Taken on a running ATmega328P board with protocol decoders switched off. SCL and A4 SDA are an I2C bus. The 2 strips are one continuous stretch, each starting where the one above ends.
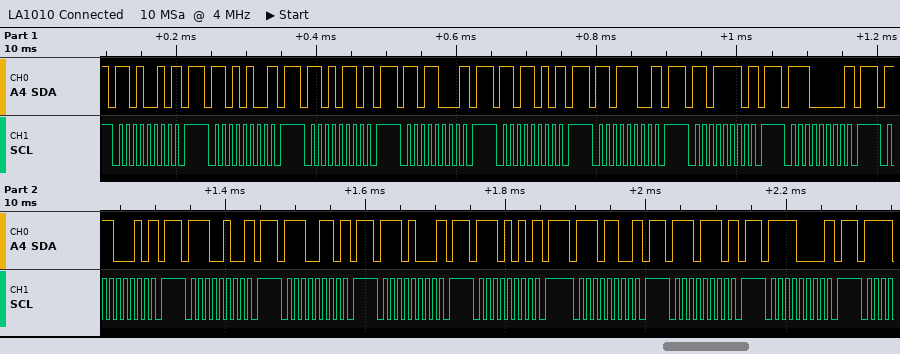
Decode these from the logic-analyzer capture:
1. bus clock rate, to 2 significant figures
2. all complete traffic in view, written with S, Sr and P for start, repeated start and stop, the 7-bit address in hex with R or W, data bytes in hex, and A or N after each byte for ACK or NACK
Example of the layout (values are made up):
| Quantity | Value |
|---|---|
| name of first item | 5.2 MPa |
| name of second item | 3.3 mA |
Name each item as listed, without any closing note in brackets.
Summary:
| Quantity | Value |
|---|---|
| bus clock rate, to 2 significant figures | 100 kHz |
| all complete traffic in view, written with S, Sr and P for start, repeated start and stop, the 7-bit address in hex with R or W, data bytes in hex, and A or N after each byte for ACK or NACK | S 69W N P S 6AW N P S 6BW N P S 6CW N P S 6DW N P S 6EW N P S 6FW N P S 70W N P S 71W N P S 72W N P S 73W N P S 74W N P S 75W N P S 76W N P S 77W N P S 78W N P |
